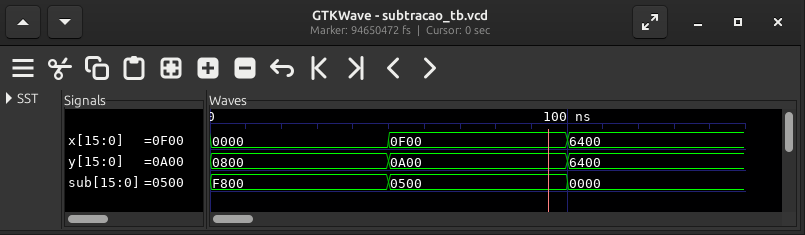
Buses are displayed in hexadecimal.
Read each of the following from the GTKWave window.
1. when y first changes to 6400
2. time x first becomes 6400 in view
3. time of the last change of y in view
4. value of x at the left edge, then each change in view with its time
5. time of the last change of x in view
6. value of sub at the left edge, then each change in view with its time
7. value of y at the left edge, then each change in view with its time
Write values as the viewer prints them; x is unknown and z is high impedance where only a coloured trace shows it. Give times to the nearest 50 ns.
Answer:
100 ns
100 ns
100 ns
0000, 0F00 at 50 ns, 6400 at 100 ns
100 ns
F800, 0500 at 50 ns, 0000 at 100 ns
0800, 0A00 at 50 ns, 6400 at 100 ns
